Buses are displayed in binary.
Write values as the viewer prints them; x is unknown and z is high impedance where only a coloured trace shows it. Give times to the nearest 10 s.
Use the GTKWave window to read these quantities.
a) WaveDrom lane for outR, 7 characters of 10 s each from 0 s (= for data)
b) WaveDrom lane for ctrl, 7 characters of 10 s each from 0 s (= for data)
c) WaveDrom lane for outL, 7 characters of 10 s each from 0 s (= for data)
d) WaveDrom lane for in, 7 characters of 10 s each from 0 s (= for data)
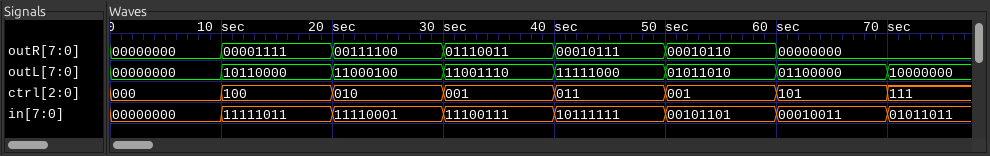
{name: 'outR', wave: '=======', data: '00000000 00001111 00111100 01110011 00010111 00010110 00000000'}
{name: 'ctrl', wave: '=======', data: '000 100 010 001 011 001 101'}
{name: 'outL', wave: '=======', data: '00000000 10110000 11000100 11001110 11111000 01011010 01100000'}
{name: 'in', wave: '=======', data: '00000000 11111011 11110001 11100111 10111111 00101101 00010011'}
